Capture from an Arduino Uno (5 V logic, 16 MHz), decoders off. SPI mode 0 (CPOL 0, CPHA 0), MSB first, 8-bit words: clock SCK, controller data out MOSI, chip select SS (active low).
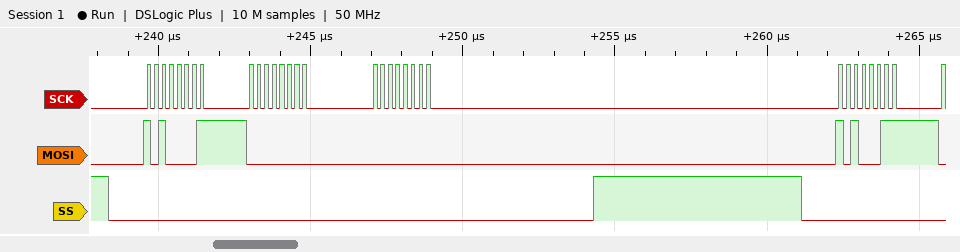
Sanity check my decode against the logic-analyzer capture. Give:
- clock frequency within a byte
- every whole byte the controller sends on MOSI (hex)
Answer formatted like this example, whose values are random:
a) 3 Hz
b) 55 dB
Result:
a) 4 MHz
b) 0xA1 0x00 0x00 0xA3
